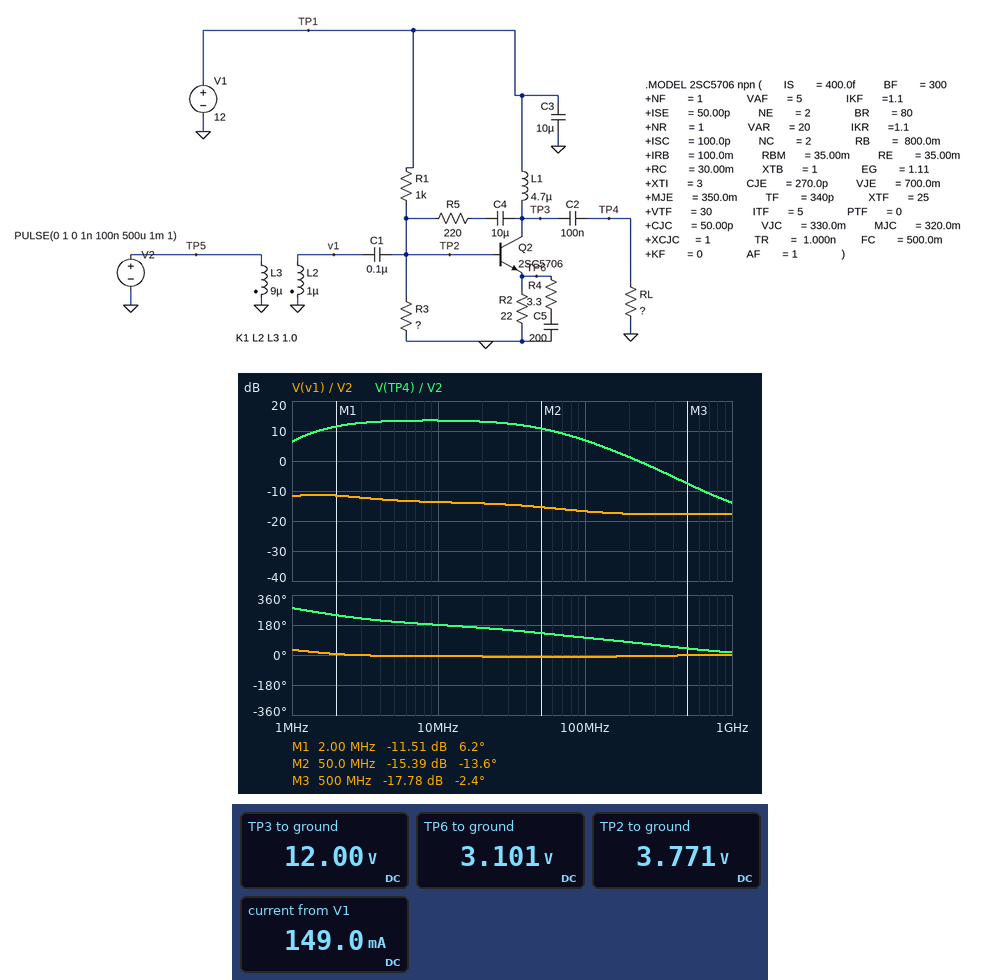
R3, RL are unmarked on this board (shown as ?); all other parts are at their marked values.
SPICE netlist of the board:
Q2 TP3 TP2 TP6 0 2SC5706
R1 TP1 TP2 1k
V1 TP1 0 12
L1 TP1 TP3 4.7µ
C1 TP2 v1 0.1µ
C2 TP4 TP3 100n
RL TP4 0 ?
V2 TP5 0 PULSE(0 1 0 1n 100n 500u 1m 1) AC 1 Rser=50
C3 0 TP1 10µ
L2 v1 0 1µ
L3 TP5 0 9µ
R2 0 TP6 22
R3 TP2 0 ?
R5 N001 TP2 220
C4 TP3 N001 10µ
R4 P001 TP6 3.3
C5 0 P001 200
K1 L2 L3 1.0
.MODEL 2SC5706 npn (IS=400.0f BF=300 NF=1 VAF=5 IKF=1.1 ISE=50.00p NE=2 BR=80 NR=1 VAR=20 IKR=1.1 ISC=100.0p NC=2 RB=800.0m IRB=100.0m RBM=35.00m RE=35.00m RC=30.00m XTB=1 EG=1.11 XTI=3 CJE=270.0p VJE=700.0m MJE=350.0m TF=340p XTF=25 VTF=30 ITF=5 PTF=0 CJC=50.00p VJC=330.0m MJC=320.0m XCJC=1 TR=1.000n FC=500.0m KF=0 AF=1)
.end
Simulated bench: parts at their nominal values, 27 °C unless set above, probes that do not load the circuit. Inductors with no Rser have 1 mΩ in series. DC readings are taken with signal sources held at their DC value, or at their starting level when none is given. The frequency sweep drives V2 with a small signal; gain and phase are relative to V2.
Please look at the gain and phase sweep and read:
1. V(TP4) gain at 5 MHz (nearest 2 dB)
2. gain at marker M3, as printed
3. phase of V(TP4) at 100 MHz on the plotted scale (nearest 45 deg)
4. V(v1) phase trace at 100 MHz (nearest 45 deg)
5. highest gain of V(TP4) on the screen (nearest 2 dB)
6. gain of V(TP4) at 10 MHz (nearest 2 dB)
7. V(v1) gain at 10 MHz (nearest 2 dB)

14 dB
-17.78 dB
90 deg
0 deg
14 dB
14 dB
-14 dB
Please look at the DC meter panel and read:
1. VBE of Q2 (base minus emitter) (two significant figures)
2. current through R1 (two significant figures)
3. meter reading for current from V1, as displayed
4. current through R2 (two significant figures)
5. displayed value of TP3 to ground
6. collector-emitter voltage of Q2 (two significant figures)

670 mV
8.2 mA
149.0 mA
140 mA
12.00 V
8.9 V
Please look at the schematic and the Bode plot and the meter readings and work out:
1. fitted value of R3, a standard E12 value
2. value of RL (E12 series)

470 Ω
120 Ω
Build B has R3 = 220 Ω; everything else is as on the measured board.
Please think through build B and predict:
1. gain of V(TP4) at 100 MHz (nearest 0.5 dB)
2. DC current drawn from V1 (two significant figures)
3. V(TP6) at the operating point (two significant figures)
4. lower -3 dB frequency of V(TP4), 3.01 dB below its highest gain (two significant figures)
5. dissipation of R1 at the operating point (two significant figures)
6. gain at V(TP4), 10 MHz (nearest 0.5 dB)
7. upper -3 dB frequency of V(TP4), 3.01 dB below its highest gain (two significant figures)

6.5 dB
78 mA
1.5 V
1.7 MHz
97 mW
13.0 dB
56 MHz
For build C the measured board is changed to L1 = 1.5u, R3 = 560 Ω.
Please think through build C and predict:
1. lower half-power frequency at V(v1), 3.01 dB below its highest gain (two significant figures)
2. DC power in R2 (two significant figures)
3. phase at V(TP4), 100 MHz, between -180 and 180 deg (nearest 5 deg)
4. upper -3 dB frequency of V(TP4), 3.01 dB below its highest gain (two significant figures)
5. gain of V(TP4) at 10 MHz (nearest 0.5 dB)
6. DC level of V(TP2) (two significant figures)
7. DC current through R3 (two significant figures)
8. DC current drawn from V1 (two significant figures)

730 kHz
570 mW
105 deg
57 MHz
13.0 dB
4.2 V
7.5 mA
170 mA
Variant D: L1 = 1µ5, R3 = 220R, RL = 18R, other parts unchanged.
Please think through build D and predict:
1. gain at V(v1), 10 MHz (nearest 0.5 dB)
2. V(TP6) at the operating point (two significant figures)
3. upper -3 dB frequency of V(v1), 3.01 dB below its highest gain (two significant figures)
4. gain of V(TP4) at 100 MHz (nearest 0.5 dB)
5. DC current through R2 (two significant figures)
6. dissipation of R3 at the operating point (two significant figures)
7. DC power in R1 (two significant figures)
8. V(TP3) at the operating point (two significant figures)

-11.0 dB
1.5 V
100 MHz
-1.0 dB
68 mA
21 mW
97 mW
12 V
